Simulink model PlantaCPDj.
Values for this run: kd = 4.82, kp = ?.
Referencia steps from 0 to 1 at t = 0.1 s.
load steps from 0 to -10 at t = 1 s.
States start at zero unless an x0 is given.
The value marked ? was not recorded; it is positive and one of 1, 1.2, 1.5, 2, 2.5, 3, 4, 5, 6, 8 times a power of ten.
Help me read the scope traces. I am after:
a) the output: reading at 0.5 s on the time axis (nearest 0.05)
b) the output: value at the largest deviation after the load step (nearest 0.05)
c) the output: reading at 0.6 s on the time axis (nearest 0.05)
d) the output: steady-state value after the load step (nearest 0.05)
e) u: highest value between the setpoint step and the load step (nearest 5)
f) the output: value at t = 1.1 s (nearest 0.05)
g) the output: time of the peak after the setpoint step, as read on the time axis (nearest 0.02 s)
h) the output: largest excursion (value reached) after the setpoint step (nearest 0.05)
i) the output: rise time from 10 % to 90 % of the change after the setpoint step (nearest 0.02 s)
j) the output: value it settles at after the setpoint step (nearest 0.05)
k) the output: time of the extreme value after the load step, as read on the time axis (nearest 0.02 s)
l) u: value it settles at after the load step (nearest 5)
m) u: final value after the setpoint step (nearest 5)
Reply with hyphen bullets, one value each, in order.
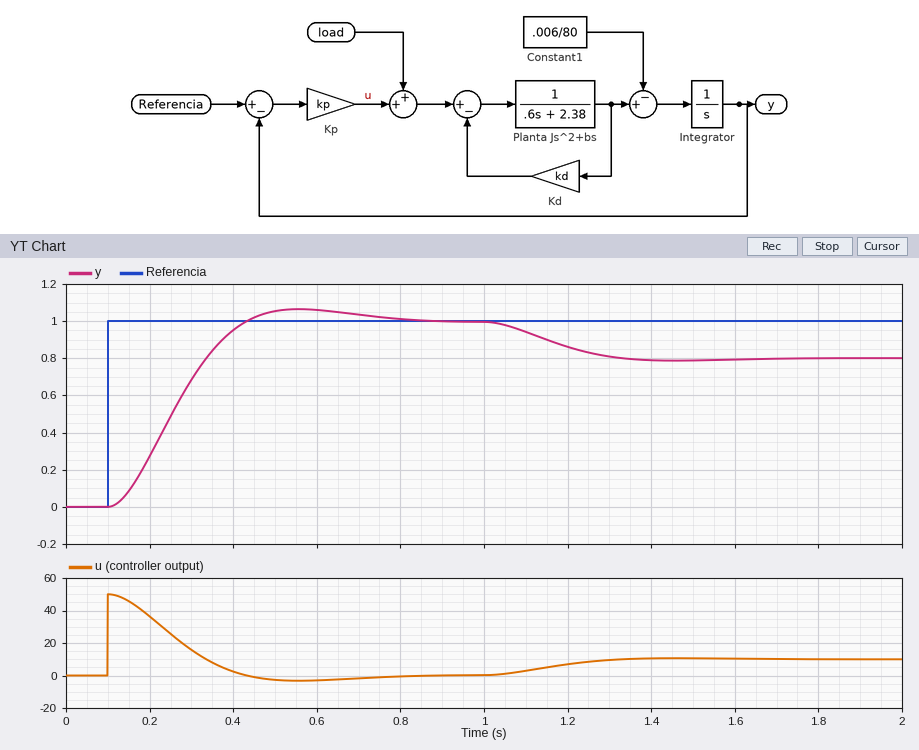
- 1.05
- 0.80
- 1.05
- 0.80
- 50
- 0.95
- 0.56 s
- 1.05
- 0.22 s
- 1.00
- 1.46 s
- 10
- 0
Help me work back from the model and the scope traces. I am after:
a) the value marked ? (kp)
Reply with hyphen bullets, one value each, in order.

- 50
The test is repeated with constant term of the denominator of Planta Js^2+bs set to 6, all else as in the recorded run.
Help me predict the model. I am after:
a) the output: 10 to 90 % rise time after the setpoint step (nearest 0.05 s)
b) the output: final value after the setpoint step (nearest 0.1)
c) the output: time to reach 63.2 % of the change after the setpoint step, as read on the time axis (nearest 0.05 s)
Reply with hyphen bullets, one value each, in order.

- 0.35 s
- 1.0
- 0.35 s
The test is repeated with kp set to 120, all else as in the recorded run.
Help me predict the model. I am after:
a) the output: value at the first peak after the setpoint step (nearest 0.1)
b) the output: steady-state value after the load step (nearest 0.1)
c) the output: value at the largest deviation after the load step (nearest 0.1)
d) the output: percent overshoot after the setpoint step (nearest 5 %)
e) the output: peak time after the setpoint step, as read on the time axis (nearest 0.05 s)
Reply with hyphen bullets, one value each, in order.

- 1.2
- 0.9
- 0.9
- 25 %
- 0.35 s
